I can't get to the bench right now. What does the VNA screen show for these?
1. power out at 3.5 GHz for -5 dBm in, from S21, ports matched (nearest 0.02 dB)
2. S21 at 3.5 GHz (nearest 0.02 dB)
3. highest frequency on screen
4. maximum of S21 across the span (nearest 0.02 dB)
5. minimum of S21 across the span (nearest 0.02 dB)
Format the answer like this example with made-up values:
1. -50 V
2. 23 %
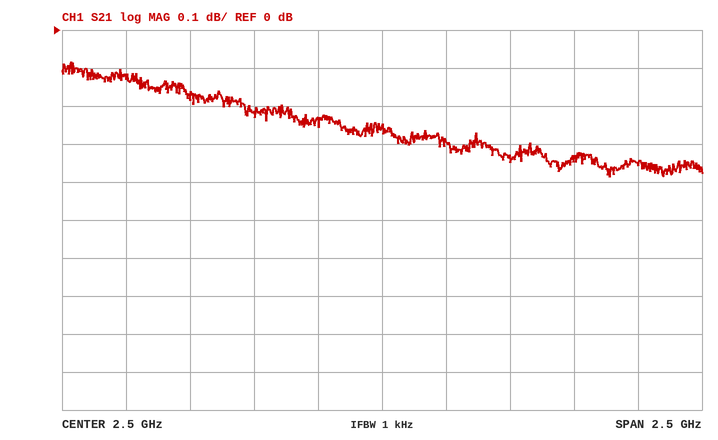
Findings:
1. -5.36 dBm
2. -0.36 dB
3. 3.75 GHz
4. -0.08 dB
5. -0.38 dB
